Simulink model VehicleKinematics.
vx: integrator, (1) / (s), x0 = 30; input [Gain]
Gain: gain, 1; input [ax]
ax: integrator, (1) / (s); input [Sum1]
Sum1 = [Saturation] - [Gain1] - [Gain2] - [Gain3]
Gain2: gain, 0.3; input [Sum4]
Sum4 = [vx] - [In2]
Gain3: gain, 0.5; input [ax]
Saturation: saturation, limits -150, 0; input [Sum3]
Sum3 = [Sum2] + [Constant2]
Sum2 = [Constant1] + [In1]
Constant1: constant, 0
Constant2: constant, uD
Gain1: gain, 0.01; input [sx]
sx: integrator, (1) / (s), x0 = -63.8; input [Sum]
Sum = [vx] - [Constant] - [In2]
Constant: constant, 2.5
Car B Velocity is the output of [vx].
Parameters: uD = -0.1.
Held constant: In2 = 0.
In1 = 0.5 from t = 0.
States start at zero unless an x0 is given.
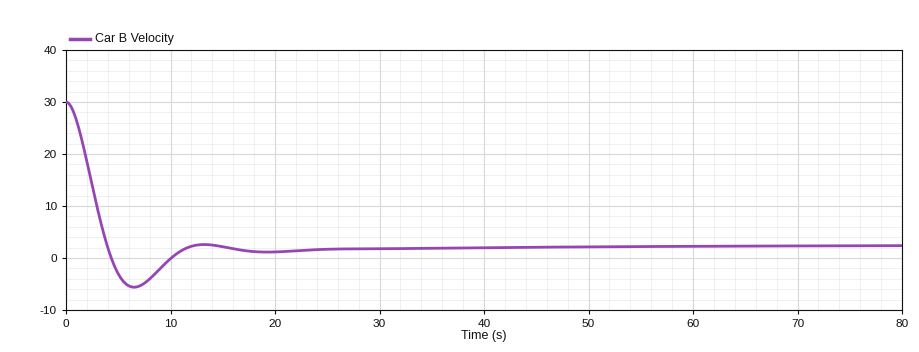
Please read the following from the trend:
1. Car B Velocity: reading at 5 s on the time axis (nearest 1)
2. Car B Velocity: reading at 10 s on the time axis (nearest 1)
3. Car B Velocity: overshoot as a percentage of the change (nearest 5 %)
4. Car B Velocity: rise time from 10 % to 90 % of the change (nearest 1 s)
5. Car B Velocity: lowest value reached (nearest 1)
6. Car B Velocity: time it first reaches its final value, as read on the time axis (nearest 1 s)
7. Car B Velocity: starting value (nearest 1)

-3
0
30 %
3 s
-6
4 s
30
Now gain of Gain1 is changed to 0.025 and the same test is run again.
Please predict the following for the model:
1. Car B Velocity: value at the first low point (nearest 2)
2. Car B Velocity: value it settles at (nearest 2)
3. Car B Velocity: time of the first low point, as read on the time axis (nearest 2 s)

-6
2
6 s
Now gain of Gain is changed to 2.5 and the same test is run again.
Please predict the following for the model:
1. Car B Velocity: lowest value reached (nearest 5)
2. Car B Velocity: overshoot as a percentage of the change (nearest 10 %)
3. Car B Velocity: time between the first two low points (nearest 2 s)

-10
50 %
8 s
